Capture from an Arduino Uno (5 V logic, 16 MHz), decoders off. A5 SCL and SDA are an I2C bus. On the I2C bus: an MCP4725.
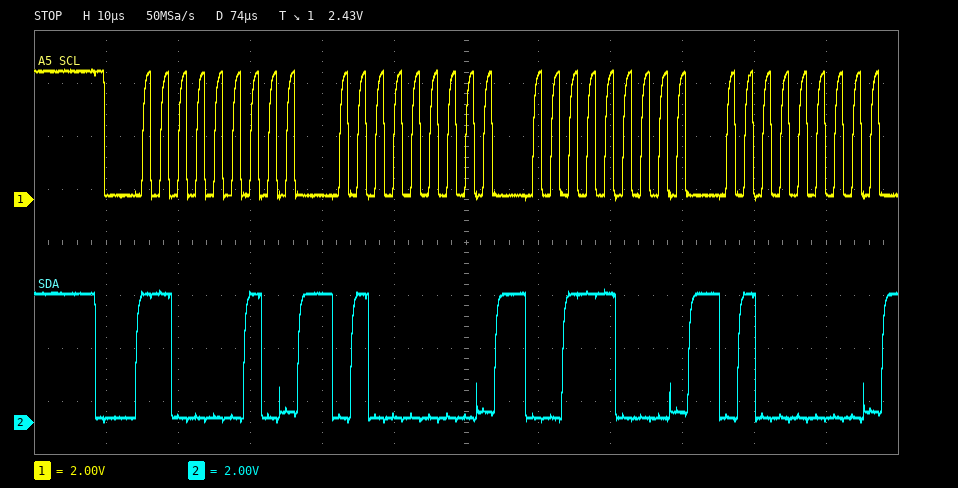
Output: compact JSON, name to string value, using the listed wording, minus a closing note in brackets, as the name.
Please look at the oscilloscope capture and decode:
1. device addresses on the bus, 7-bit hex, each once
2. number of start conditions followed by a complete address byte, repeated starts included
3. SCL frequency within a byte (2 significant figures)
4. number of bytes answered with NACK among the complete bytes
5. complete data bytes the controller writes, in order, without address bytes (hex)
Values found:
{"device addresses on the bus, 7-bit hex, each once": "0x61", "number of start conditions followed by a complete address byte, repeated starts included": "1", "SCL frequency within a byte": "400 kHz", "number of bytes answered with NACK among the complete bytes": "0", "complete data bytes the controller writes, in order, without address bytes": "40 38 40"}
